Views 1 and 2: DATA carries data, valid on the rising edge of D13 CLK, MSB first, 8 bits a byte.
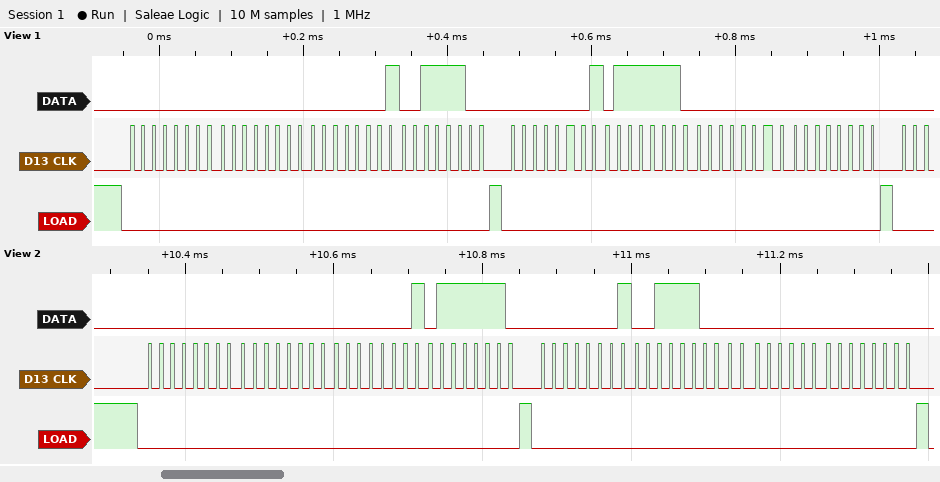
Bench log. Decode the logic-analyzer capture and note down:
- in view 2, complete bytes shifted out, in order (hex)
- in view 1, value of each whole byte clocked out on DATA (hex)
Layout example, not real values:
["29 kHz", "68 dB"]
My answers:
["00 00 01 7E 01 3C 00 00", "00 00 01 3C 01 7E 00 00"]
